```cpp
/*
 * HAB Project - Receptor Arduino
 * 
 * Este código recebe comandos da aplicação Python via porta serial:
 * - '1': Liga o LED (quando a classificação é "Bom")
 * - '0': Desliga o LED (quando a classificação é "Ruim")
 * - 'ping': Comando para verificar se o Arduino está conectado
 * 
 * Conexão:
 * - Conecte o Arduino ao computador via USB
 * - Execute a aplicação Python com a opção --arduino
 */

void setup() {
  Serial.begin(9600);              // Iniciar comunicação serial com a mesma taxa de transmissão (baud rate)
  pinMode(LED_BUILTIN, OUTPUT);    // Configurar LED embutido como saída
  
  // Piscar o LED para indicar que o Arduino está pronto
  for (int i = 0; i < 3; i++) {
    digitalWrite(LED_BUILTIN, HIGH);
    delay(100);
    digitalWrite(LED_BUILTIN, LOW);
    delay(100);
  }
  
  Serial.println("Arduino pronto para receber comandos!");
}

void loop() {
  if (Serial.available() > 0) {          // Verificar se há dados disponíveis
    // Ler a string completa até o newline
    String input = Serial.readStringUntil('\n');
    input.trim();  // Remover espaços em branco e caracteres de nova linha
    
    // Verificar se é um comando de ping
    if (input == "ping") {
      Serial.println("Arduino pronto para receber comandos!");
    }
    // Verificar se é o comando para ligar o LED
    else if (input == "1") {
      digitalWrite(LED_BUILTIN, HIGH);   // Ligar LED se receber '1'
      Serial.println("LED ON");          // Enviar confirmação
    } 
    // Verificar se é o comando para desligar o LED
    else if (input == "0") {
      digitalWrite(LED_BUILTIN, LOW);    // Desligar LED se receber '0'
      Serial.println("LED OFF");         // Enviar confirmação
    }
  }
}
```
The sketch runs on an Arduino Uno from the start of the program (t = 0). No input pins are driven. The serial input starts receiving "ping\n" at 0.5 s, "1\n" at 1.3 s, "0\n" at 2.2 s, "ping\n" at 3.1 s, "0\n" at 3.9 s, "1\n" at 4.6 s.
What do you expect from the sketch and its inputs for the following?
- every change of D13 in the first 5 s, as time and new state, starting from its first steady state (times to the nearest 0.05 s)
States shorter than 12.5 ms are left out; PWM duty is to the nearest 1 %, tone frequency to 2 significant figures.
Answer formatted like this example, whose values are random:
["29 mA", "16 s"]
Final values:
["0 s high; 0.1 s low; 0.2 s high; 0.3 s low; 0.4 s high; 0.5 s low; 1.3 s high; 2.2 s low; 4.6 s high"]
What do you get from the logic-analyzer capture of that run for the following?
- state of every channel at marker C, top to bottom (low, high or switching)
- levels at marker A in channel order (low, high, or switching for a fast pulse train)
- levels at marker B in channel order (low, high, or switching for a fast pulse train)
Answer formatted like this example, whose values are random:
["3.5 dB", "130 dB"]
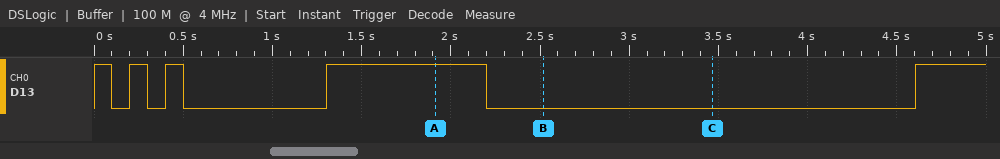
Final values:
["D13 low", "D13 high", "D13 low"]
